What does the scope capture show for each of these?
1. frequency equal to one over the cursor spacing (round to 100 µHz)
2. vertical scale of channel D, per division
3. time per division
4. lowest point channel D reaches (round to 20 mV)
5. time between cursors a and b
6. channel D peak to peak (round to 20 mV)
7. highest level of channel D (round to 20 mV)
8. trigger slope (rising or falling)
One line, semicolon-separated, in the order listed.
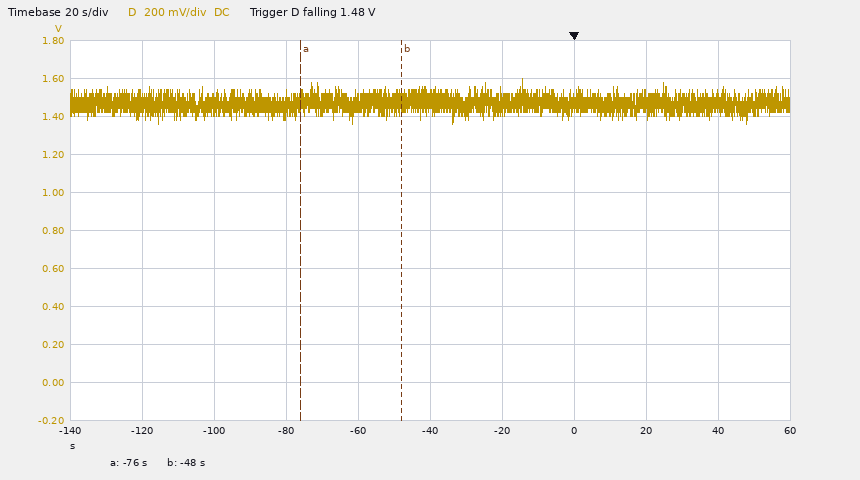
35.7 mHz; 200 mV; 20 s; 1.36 V; 28 s; 240 mV; 1.60 V; falling
